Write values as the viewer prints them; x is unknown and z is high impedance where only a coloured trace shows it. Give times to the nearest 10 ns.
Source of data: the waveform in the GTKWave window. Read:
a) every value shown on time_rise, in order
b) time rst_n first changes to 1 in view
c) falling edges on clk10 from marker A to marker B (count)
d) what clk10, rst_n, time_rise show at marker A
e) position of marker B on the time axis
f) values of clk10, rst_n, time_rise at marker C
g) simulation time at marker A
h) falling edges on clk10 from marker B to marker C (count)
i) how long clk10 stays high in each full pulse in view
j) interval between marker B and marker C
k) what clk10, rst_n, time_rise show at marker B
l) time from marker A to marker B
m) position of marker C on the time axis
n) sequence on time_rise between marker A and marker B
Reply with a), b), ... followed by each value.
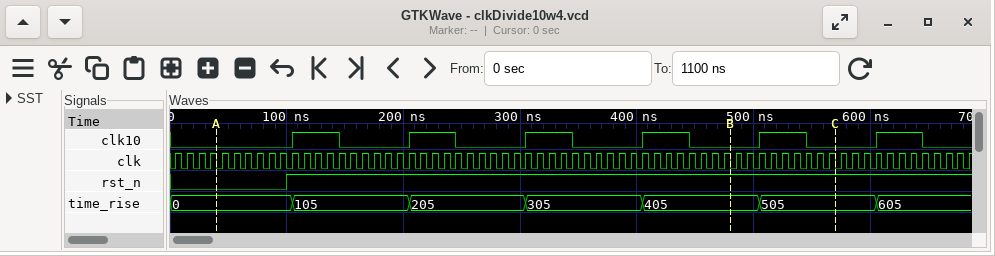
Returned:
a) 0, 105, 205, 305, 405, 505, 605
b) 100 ns
c) 4
d) clk10=0, rst_n=0, time_rise=0
e) 480 ns
f) clk10=0, rst_n=1, time_rise=505
g) 40 ns
h) 1
i) 40 ns, 40 ns, 40 ns, 40 ns, 40 ns, 40 ns
j) 90 ns
k) clk10=0, rst_n=1, time_rise=405
l) 440 ns
m) 570 ns
n) 0, 105, 205, 305, 405
